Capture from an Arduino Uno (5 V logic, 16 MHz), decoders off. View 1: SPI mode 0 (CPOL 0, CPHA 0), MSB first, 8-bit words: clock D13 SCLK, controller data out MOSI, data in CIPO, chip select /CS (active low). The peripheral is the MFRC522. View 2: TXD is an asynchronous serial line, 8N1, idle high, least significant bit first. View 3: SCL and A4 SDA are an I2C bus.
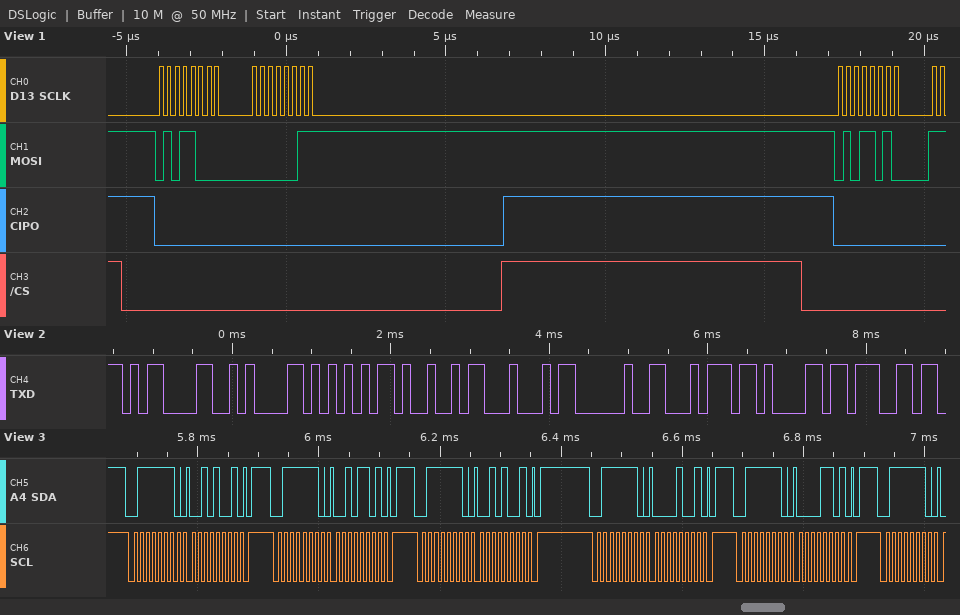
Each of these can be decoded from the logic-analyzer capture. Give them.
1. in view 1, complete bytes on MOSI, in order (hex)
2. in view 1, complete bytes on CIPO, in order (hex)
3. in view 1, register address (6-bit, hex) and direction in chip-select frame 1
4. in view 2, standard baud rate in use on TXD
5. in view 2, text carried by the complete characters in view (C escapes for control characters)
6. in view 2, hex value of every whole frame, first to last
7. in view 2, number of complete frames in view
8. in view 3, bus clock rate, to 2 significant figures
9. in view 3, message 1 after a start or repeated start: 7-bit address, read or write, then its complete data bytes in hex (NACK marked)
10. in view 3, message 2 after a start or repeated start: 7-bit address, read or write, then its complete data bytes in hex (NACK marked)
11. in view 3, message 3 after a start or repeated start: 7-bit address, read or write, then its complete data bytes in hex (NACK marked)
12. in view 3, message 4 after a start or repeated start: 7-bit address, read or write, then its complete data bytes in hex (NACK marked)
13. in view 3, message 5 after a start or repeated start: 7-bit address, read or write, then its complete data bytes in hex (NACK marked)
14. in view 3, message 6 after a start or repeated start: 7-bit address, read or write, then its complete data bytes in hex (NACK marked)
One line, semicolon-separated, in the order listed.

0x58 0x03 0x5A; 0x00 0x00 0x00; 0x2C write; 9600 baud; "\r\nUID tag"; 0x0D 0x0A 0x55 0x49 0x44 0x20 0x74 0x61 0x67; 9; 100 kHz; 0x3F write: 29; 0x3F write: 2D; 0x3F write: 29; 0x3F write: 09; 0x3F write: 0D; 0x3F write
